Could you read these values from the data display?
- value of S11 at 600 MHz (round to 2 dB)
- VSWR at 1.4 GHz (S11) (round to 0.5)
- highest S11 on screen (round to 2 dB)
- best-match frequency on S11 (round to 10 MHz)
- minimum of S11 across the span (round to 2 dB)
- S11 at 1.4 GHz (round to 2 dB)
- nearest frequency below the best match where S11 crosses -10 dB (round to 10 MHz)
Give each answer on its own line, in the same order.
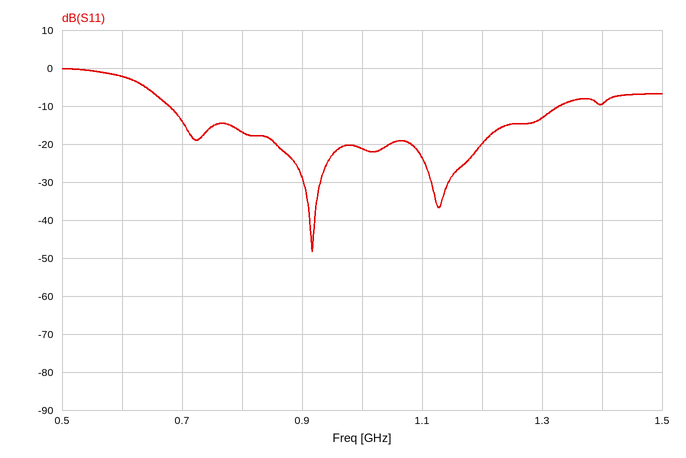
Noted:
-2 dB
2.0
0 dB
920 MHz
-48 dB
-10 dB
680 MHz
